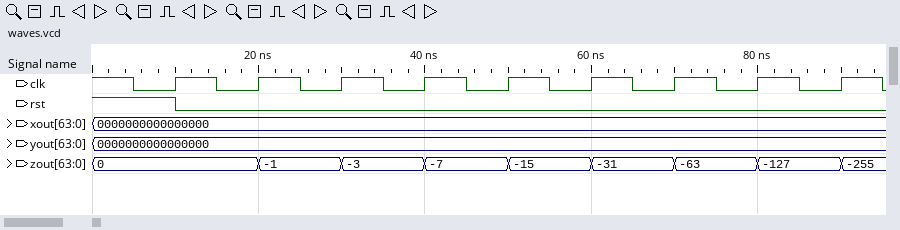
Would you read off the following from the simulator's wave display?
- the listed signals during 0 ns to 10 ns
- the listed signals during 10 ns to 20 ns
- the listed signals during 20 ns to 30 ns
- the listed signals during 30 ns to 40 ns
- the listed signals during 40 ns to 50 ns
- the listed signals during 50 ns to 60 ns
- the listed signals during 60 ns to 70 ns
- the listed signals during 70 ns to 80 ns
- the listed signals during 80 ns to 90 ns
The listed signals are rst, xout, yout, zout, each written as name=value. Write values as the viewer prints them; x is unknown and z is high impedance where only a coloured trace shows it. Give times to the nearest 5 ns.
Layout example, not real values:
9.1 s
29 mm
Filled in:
rst=1, xout=0000000000000000, yout=0000000000000000, zout=0
rst=0, xout=0000000000000000, yout=0000000000000000, zout=0
rst=0, xout=0000000000000000, yout=0000000000000000, zout=-1
rst=0, xout=0000000000000000, yout=0000000000000000, zout=-3
rst=0, xout=0000000000000000, yout=0000000000000000, zout=-7
rst=0, xout=0000000000000000, yout=0000000000000000, zout=-15
rst=0, xout=0000000000000000, yout=0000000000000000, zout=-31
rst=0, xout=0000000000000000, yout=0000000000000000, zout=-63
rst=0, xout=0000000000000000, yout=0000000000000000, zout=-127
